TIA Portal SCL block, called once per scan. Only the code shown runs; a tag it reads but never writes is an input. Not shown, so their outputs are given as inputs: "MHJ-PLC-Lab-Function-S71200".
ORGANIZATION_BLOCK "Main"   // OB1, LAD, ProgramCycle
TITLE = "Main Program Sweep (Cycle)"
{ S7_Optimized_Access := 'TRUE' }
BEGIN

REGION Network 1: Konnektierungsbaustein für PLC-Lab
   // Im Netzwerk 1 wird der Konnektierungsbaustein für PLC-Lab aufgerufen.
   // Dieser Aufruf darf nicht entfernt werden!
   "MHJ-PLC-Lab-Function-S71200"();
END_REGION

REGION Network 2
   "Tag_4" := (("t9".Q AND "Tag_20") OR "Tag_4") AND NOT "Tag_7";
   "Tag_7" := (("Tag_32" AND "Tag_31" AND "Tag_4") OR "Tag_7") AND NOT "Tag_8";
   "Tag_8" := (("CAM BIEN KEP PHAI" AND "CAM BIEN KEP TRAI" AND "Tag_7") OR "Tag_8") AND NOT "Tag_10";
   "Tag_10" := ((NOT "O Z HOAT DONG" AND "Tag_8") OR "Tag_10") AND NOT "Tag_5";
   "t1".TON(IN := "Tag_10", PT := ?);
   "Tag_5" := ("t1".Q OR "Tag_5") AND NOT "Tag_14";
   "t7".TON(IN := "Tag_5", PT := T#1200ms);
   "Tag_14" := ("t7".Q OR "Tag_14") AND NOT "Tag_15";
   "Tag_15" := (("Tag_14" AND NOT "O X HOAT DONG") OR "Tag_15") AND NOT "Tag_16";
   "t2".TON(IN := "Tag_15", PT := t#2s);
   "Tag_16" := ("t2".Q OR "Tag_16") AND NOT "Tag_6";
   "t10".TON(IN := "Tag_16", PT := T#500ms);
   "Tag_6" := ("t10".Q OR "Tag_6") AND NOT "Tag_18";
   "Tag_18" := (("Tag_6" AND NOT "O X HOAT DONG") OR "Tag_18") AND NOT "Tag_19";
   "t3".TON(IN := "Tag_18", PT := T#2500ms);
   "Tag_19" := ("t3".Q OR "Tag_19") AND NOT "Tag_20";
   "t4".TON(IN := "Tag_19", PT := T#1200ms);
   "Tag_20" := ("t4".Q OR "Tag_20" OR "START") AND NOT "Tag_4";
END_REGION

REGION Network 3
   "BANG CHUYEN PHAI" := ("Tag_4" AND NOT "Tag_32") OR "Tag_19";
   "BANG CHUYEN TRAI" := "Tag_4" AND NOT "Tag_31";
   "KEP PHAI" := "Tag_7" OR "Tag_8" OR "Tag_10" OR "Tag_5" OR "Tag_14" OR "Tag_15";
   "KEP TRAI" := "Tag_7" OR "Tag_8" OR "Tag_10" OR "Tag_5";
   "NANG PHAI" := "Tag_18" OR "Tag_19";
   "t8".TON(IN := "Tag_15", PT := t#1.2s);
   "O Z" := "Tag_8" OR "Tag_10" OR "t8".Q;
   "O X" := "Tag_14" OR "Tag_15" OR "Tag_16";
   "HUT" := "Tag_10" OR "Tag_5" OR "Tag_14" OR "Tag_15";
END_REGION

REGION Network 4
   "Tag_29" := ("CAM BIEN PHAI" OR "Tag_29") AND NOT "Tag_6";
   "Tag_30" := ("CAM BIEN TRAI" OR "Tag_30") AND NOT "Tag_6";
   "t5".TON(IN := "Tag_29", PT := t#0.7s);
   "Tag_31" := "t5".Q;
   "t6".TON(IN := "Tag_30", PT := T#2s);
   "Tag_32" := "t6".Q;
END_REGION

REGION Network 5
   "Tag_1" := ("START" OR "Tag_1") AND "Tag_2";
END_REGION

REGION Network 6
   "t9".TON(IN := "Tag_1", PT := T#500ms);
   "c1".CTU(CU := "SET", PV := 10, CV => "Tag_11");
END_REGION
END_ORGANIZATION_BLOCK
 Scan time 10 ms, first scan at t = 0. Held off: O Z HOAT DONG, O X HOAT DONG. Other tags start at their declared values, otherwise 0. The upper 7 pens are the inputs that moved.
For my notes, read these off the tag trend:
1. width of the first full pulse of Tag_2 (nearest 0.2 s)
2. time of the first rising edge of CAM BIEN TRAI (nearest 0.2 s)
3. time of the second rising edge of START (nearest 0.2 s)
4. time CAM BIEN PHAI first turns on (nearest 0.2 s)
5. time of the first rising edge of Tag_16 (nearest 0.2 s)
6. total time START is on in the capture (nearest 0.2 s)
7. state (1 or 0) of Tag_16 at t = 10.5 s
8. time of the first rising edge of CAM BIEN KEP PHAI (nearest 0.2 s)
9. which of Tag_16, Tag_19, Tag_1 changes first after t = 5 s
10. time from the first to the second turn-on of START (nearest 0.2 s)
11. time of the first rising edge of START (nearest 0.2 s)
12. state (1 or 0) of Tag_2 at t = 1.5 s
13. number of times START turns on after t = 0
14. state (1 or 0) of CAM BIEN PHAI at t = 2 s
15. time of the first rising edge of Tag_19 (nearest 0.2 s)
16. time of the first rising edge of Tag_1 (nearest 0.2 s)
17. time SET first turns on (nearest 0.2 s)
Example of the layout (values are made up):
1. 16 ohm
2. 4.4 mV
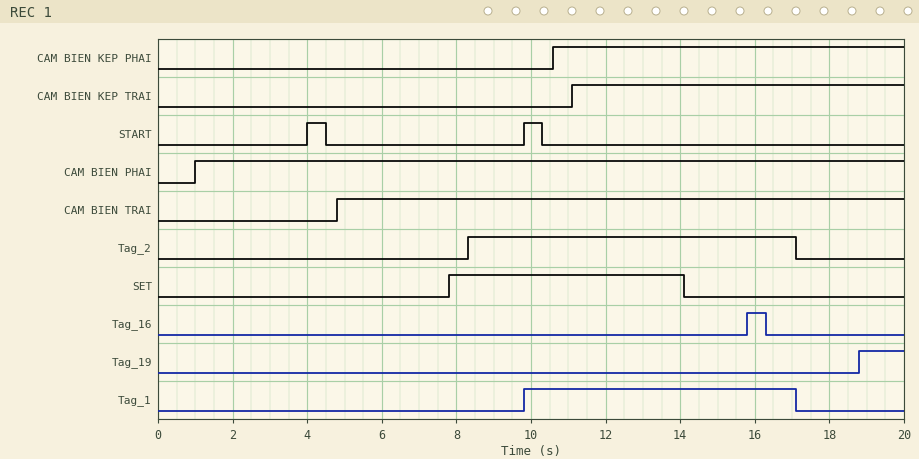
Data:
1. 8.8 s
2. 4.8 s
3. 9.8 s
4. 1.0 s
5. 15.8 s
6. 1.0 s
7. 0
8. 10.6 s
9. Tag_1
10. 5.8 s
11. 4.0 s
12. 0
13. 2
14. 1
15. 18.8 s
16. 9.8 s
17. 7.8 s
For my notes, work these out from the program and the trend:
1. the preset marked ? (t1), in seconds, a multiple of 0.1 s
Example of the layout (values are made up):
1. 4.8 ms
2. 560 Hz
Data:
1. 1.5 s
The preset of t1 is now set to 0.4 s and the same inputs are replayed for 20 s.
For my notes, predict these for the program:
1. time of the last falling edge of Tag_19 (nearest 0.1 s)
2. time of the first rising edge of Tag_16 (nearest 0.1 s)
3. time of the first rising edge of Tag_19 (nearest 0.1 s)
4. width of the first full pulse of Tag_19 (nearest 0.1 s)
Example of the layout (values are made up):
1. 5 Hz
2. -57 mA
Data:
1. 18.9 s
2. 14.7 s
3. 17.7 s
4. 1.2 s
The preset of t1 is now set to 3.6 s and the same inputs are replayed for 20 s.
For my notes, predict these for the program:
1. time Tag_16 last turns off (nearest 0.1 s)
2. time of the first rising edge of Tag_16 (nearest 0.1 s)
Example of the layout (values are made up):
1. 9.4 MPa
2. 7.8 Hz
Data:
1. 18.4 s
2. 17.9 s
